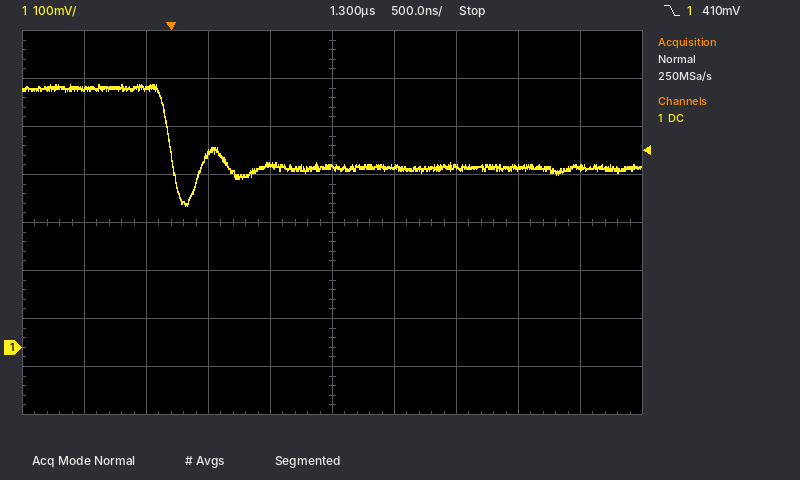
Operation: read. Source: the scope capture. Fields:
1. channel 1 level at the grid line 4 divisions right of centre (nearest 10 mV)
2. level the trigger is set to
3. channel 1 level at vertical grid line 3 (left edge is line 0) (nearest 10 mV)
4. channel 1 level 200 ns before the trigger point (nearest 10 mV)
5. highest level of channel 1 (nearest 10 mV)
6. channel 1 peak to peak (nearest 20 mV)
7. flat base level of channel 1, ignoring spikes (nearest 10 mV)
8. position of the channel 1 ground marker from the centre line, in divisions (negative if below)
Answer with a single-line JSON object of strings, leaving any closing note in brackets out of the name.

{"channel 1 level at the grid line 4 divisions right of centre": "370 mV", "level the trigger is set to": "410 mV", "channel 1 level at vertical grid line 3 (left edge is line 0)": "400 mV", "channel 1 level 200 ns before the trigger point": "540 mV", "highest level of channel 1": "550 mV", "channel 1 peak to peak": "260 mV", "flat base level of channel 1, ignoring spikes": "370 mV", "position of the channel 1 ground marker from the centre line, in divisions": "-2.6 div"}
